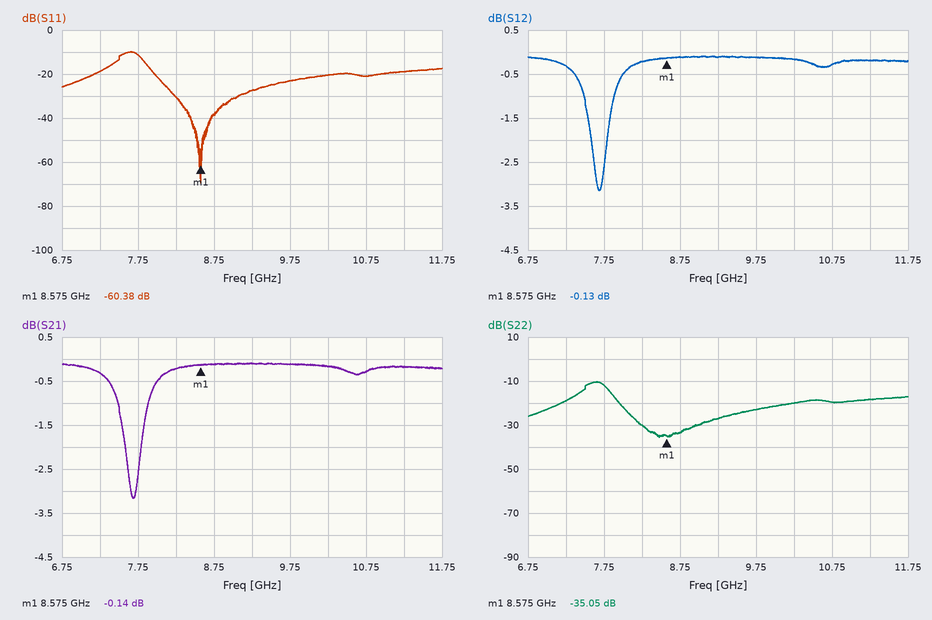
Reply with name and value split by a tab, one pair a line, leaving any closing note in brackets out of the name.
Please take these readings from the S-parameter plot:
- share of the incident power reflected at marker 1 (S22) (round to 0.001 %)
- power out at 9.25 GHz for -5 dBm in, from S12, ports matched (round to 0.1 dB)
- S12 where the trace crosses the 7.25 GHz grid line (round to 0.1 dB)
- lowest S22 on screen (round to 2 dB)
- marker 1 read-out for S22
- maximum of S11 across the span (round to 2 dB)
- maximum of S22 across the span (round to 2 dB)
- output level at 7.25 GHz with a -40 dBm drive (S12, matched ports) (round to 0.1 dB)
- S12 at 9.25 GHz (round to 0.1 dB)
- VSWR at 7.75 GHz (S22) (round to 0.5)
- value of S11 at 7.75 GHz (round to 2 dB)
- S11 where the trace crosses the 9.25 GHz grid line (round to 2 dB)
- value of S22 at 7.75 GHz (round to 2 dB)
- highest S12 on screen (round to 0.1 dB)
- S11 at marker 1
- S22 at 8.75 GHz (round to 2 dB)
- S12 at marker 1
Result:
share of the incident power reflected at marker 1 (S22)	0.031 %
power out at 9.25 GHz for -5 dBm in, from S12, ports matched	-5.1 dBm
S12 where the trace crosses the 7.25 GHz grid line	-0.3 dB
lowest S22 on screen	-36 dB
marker 1 read-out for S22	-35.05 dB
maximum of S11 across the span	-10 dB
maximum of S22 across the span	-10 dB
output level at 7.25 GHz with a -40 dBm drive (S12, matched ports)	-40.3 dBm
S12 at 9.25 GHz	-0.1 dB
VSWR at 7.75 GHz (S22)	1.5
value of S11 at 7.75 GHz	-12 dB
S11 where the trace crosses the 9.25 GHz grid line	-28 dB
value of S22 at 7.75 GHz	-12 dB
highest S12 on screen	-0.1 dB
S11 at marker 1	-60.38 dB
S22 at 8.75 GHz	-34 dB
S12 at marker 1	-0.13 dB
